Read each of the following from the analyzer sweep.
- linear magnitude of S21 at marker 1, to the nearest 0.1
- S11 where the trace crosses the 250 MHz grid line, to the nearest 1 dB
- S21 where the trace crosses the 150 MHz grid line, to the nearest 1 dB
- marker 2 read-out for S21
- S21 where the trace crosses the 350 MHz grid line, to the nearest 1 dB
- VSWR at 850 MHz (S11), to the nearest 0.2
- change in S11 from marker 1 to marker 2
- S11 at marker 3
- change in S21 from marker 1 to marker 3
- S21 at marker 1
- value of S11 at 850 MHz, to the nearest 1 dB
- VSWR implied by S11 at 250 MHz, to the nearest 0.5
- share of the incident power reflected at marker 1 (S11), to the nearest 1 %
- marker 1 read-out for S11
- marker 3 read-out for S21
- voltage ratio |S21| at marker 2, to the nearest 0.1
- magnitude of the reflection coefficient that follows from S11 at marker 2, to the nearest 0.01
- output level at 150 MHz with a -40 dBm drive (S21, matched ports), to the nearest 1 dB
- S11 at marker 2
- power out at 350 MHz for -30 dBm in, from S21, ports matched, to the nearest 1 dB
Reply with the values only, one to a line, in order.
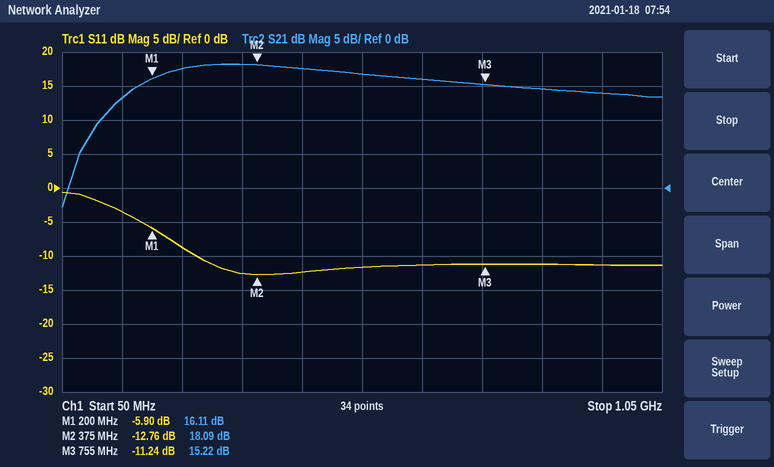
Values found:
6.4
-9 dB
13 dB
18.09 dB
18 dB
1.8
-6.86 dB
-11.24 dB
-0.89 dB
16.11 dB
-11 dB
2.0
26 %
-5.90 dB
15.22 dB
8.0
0.23
-27 dBm
-12.76 dB
-12 dBm
